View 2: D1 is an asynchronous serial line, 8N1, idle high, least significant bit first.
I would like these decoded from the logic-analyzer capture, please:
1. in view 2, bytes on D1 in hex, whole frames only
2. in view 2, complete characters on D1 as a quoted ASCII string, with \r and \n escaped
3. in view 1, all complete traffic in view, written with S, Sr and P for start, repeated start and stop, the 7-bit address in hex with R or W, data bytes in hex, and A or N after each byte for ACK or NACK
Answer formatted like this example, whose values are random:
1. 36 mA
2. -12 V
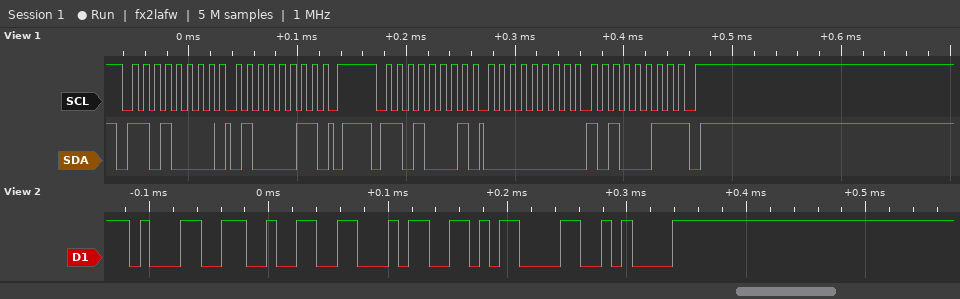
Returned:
1. 31 32 34 0D 0A
2. "124\r\n"
3. S 68W A 43 A P S 68R A 00 A A3 N P
